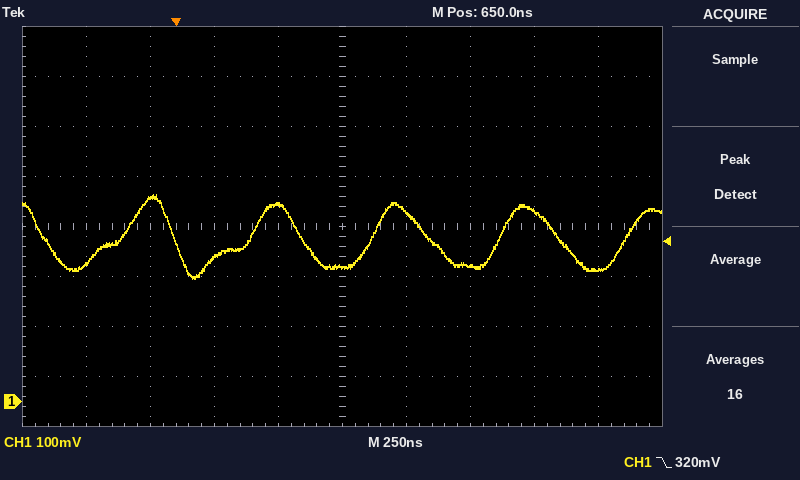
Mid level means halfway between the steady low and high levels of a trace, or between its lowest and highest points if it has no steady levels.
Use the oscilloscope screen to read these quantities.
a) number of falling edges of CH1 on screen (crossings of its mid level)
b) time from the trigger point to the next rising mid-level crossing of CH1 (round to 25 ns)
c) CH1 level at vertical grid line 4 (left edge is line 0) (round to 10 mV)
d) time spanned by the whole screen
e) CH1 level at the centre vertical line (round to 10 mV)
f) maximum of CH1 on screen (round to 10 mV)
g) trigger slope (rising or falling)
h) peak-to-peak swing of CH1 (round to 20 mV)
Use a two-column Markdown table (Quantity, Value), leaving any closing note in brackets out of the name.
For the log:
| Quantity | Value |
|---|---|
| number of falling edges of CH1 on screen | 5 |
| time from the trigger point to the next rising mid-level crossing of CH1 | 300 ns |
| CH1 level at vertical grid line 4 (left edge is line 0) | 390 mV |
| time spanned by the whole screen | 2.5 µs |
| CH1 level at the centre vertical line | 270 mV |
| maximum of CH1 on screen | 410 mV |
| trigger slope | falling |
| peak-to-peak swing of CH1 | 160 mV |
